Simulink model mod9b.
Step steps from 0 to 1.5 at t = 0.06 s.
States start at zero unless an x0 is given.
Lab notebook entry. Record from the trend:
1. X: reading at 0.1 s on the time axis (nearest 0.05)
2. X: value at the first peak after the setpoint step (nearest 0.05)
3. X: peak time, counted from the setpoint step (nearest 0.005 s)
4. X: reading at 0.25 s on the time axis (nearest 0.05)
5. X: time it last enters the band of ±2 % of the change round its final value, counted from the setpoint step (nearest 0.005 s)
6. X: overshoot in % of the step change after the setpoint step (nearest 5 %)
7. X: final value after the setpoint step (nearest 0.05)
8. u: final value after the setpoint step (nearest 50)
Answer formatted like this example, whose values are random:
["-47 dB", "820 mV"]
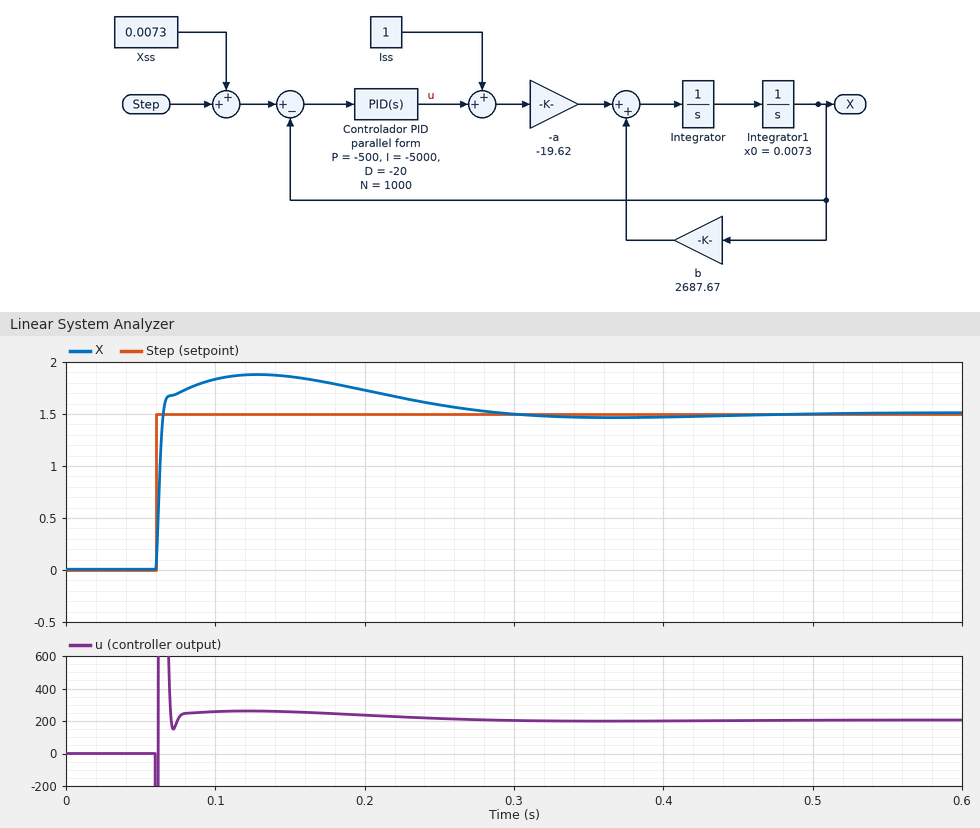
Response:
["1.85", "1.90", "0.070 s", "1.60", "0.365 s", "25 %", "1.50", "200"]
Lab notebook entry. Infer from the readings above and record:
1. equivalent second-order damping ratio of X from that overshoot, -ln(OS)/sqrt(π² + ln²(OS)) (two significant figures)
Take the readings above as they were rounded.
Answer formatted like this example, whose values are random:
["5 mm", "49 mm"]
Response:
["0.40"]
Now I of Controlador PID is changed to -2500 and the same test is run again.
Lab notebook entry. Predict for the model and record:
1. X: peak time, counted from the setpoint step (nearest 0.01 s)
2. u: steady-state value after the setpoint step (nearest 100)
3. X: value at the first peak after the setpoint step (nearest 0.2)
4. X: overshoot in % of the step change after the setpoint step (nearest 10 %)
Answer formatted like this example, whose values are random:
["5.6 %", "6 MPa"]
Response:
["0.09 s", "200", "2.0", "30 %"]
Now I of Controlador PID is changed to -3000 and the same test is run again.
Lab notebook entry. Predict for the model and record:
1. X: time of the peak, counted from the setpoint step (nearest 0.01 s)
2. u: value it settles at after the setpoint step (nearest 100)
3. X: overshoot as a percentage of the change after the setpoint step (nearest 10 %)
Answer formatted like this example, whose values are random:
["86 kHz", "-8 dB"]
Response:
["0.08 s", "200", "30 %"]
